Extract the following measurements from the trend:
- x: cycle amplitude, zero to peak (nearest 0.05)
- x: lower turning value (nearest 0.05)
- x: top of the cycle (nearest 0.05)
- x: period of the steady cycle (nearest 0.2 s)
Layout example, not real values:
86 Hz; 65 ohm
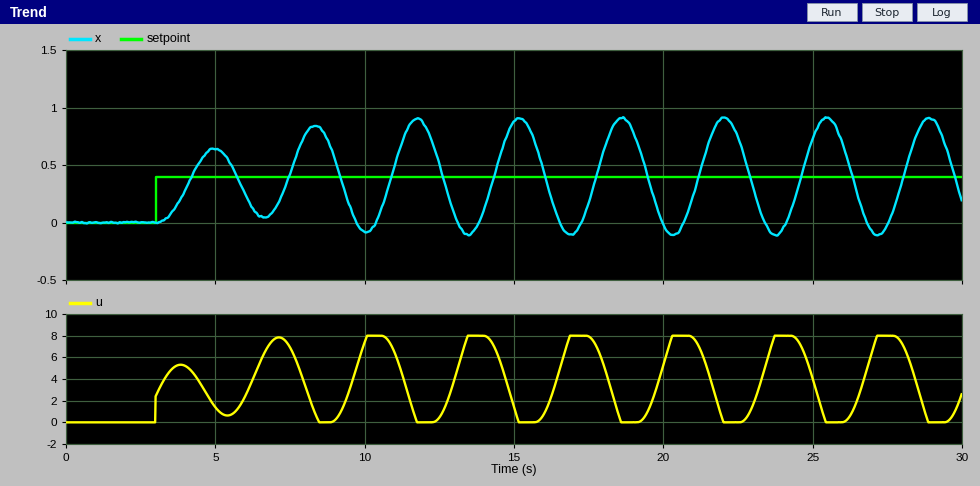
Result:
0.50; -0.10; 0.90; 3.4 s
